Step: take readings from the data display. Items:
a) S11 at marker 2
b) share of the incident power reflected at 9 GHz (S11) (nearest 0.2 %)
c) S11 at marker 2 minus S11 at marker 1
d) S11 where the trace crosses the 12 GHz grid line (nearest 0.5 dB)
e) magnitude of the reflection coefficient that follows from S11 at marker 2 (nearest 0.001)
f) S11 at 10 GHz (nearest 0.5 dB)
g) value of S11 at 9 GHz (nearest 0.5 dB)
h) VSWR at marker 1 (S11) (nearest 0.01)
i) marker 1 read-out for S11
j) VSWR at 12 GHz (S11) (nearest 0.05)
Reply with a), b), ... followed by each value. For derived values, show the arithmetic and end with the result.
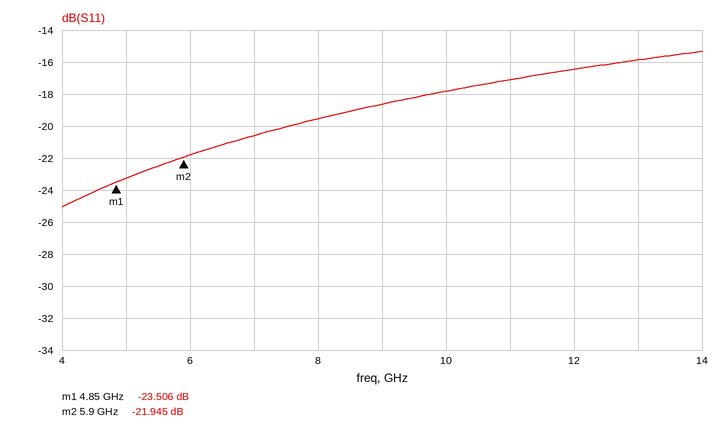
a) -21.945 dB
b) 10^(-18.5/10) ≈ 1.4 %
c) -21.945 − (-23.506) = 1.561 dB
d) -16.5 dB
e) 10^(-21.945/20) ≈ 0.080
f) -18.0 dB
g) -18.5 dB
h) (1 + 0.0668)/(1 − 0.0668) ≈ 1.14
i) -23.506 dB
j) |Γ| = 10^(-16.5/20) = 0.1496; VSWR = (1 + 0.1496)/(1 − 0.1496) ≈ 1.35
